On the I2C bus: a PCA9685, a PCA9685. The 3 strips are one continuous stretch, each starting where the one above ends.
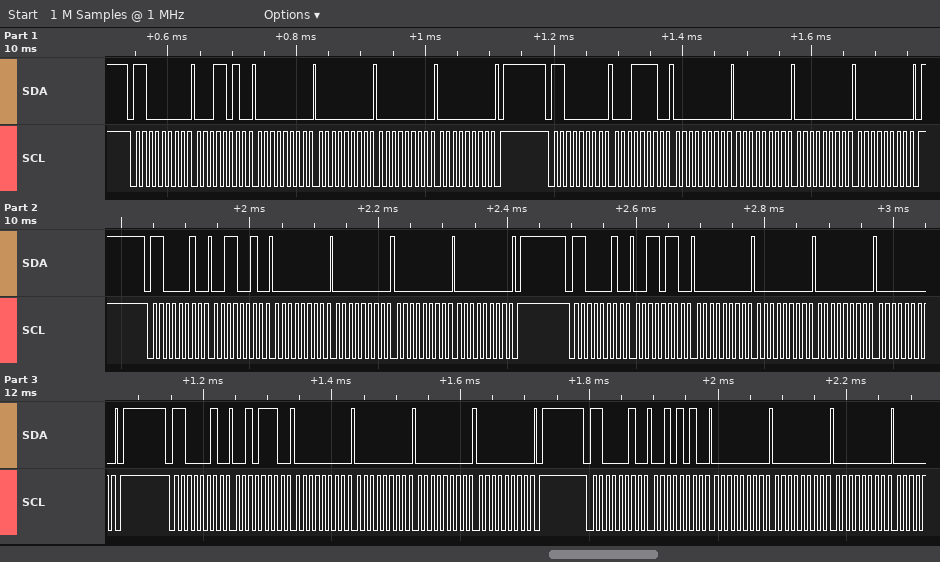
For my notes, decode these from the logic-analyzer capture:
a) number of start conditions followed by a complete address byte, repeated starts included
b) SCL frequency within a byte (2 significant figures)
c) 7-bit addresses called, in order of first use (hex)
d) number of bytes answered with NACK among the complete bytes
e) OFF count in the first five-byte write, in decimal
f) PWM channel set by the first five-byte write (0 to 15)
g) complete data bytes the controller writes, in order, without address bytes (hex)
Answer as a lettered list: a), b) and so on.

a) 6
b) 100 kHz
c) 0x60 0x61
d) 0
e) 0
f) 5
g) 1A 00 00 00 00 1E 00 00 00 00 32 00 00 00 00 36 00 00 00 00 2E 00 00 00 00 2A 00 00 00
